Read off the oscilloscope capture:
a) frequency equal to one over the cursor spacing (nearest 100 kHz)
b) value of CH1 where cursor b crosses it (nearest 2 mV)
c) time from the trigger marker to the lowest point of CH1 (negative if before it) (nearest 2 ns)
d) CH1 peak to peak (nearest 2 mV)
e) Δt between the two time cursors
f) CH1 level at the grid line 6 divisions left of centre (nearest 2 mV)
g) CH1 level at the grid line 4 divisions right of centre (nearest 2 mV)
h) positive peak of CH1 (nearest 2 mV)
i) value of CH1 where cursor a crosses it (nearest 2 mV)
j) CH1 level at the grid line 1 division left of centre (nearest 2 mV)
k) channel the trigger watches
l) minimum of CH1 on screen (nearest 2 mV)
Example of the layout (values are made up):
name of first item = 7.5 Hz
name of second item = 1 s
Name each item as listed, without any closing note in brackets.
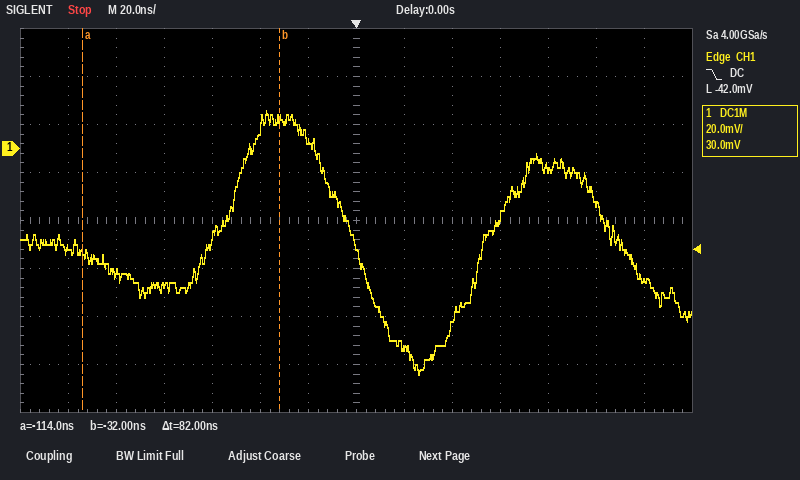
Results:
frequency equal to one over the cursor spacing = 12.2 MHz
value of CH1 where cursor b crosses it = 12 mV
time from the trigger marker to the lowest point of CH1 (negative if before it) = +26 ns
CH1 peak to peak = 110 mV
Δt between the two time cursors = 82 ns
CH1 level at the grid line 6 divisions left of centre = -42 mV
CH1 level at the grid line 4 divisions right of centre = -8 mV
positive peak of CH1 = 16 mV
value of CH1 where cursor a crosses it = -44 mV
CH1 level at the grid line 1 division left of centre = 4 mV
channel the trigger watches = CH1
minimum of CH1 on screen = -94 mV
